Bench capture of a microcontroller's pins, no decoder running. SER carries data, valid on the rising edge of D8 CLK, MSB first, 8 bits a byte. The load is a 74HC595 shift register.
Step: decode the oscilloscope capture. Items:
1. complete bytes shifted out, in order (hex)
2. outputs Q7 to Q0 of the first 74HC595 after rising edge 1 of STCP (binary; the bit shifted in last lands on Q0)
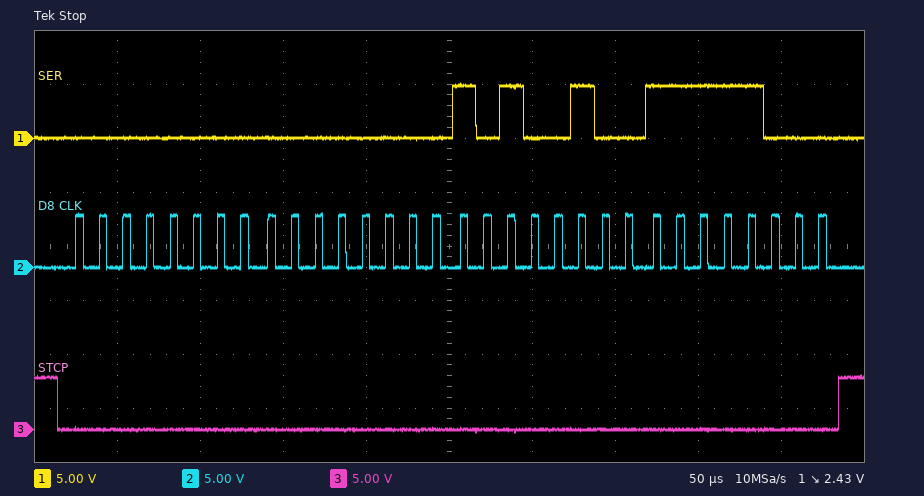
00 00 A4 F8
11111000
